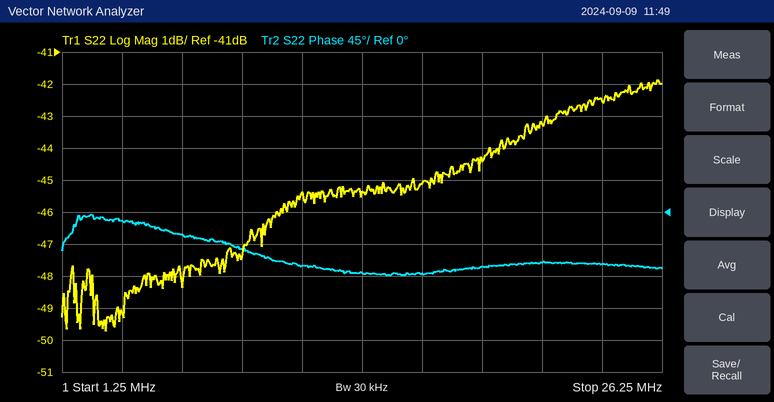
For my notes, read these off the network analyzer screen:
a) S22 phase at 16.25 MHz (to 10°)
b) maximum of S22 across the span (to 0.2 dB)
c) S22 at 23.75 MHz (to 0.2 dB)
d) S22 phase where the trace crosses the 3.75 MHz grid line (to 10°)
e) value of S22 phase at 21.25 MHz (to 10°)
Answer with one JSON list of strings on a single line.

["-90°", "-41.8 dB", "-42.6 dB", "-10°", "-70°"]
